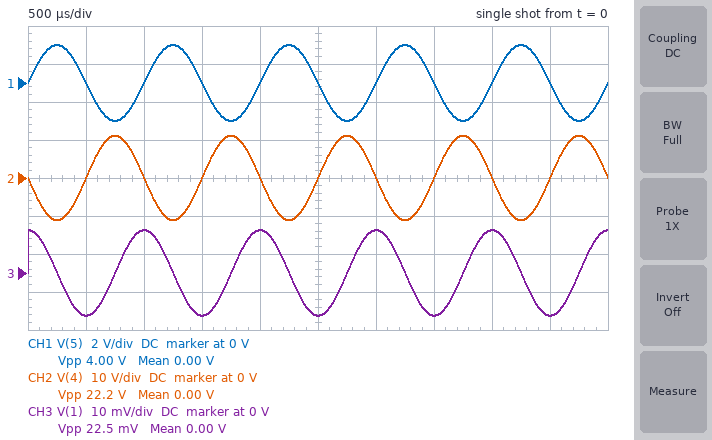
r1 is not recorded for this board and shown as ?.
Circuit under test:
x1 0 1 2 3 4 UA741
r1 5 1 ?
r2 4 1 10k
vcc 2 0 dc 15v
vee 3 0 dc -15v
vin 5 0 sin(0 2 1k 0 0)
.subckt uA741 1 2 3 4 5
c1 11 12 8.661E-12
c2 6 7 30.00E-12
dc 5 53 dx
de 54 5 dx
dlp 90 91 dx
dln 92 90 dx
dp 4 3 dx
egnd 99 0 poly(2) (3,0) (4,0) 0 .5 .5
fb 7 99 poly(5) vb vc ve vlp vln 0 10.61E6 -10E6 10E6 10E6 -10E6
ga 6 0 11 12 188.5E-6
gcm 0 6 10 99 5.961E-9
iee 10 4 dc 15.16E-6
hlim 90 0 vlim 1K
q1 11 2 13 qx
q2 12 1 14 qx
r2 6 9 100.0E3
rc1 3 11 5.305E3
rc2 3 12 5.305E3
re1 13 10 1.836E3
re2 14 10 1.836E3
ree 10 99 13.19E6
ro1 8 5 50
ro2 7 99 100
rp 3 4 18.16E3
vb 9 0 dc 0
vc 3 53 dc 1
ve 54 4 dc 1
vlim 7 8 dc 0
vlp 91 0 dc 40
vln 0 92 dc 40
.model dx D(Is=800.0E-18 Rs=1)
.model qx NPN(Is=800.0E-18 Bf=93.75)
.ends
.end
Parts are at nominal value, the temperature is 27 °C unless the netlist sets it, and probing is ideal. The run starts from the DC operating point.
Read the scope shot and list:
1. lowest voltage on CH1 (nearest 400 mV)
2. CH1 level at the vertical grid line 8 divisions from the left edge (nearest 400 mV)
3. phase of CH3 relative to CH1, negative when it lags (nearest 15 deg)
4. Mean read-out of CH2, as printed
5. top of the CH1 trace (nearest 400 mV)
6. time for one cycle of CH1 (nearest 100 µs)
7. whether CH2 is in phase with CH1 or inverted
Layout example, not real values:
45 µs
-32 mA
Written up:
-2.0 V
0 V
90 deg
0.00 V
2.0 V
1.0 ms
inverted
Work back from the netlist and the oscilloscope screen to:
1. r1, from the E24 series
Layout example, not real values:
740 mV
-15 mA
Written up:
1.8 kΩ
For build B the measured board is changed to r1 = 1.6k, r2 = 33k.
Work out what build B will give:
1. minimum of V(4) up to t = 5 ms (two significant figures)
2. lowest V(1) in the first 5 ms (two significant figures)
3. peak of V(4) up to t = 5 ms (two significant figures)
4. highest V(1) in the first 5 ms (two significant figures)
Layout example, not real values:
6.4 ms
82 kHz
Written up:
-15 V
-1.2 V
15 V
1.2 V
